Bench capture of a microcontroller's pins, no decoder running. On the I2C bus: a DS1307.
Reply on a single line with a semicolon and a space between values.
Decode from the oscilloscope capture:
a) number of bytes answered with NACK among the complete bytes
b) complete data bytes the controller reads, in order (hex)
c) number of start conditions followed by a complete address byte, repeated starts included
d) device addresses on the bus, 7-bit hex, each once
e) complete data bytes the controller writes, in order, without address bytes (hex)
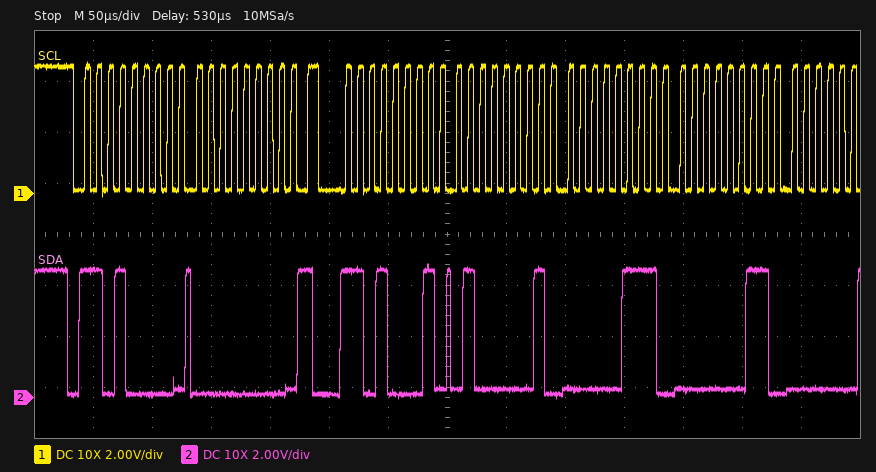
0; 41 07 03; 2; 0x68; 00
